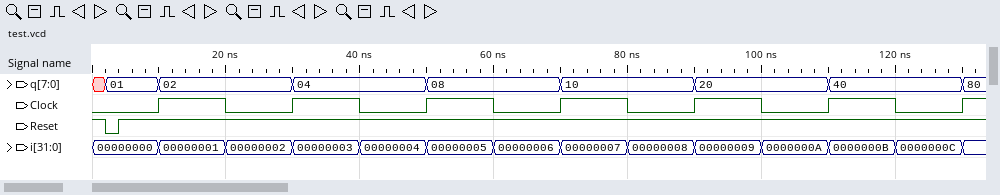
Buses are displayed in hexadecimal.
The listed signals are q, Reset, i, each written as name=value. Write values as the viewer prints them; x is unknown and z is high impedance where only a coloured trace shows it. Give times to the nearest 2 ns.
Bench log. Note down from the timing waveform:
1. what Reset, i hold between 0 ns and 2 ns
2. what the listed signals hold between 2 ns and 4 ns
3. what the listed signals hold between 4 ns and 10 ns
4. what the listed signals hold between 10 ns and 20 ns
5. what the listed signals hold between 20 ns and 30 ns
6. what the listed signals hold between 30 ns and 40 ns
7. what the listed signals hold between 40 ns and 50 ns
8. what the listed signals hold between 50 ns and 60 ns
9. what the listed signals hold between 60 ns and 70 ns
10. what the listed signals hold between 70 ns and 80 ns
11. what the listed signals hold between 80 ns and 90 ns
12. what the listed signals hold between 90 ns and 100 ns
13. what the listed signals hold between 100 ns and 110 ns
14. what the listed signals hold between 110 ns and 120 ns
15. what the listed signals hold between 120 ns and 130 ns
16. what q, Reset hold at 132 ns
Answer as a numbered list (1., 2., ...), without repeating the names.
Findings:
1. Reset=1, i=00000000
2. q=01, Reset=0, i=00000000
3. q=01, Reset=1, i=00000000
4. q=02, Reset=1, i=00000001
5. q=02, Reset=1, i=00000002
6. q=04, Reset=1, i=00000003
7. q=04, Reset=1, i=00000004
8. q=08, Reset=1, i=00000005
9. q=08, Reset=1, i=00000006
10. q=10, Reset=1, i=00000007
11. q=10, Reset=1, i=00000008
12. q=20, Reset=1, i=00000009
13. q=20, Reset=1, i=0000000A
14. q=40, Reset=1, i=0000000B
15. q=40, Reset=1, i=0000000C
16. q=80, Reset=1
